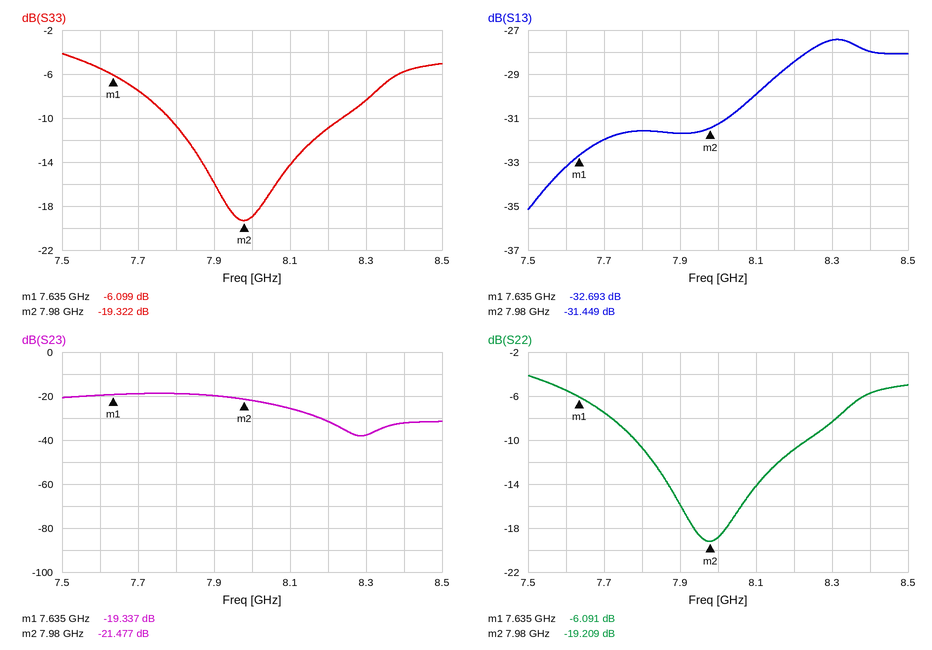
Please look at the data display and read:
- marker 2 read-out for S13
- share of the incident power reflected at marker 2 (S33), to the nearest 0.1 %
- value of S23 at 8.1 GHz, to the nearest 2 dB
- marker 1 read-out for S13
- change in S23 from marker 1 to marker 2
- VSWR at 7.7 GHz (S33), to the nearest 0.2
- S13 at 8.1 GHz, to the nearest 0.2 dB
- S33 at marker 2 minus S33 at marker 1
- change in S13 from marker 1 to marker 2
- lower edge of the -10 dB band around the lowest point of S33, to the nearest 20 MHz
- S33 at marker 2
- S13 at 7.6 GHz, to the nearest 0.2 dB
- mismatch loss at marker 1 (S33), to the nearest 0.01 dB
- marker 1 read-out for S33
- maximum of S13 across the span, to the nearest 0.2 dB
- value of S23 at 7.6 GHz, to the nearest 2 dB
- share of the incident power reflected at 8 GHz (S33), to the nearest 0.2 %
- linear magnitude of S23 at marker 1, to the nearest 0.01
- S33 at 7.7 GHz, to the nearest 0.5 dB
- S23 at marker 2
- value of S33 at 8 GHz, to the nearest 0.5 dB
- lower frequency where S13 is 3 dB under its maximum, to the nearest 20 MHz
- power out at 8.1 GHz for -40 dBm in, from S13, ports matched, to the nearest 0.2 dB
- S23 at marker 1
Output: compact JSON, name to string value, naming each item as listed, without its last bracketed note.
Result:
{"marker 2 read-out for S13": "-31.449 dB", "share of the incident power reflected at marker 2 (S33), to the nearest 0.1 %": "1.2 %", "value of S23 at 8.1 GHz, to the nearest 2 dB": "-26 dB", "marker 1 read-out for S13": "-32.693 dB", "change in S23 from marker 1 to marker 2": "-2.140 dB", "VSWR at 7.7 GHz (S33), to the nearest 0.2": "2.4", "S13 at 8.1 GHz, to the nearest 0.2 dB": "-30.0 dB", "S33 at marker 2 minus S33 at marker 1": "-13.223 dB", "change in S13 from marker 1 to marker 2": "1.244 dB", "lower edge of the -10 dB band around the lowest point of S33, to the nearest 20 MHz": "7.78 GHz", "S33 at marker 2": "-19.322 dB", "S13 at 7.6 GHz, to the nearest 0.2 dB": "-33.2 dB", "mismatch loss at marker 1 (S33), to the nearest 0.01 dB": "1.22 dB", "marker 1 read-out for S33": "-6.099 dB", "maximum of S13 across the span, to the nearest 0.2 dB": "-27.4 dB", "value of S23 at 7.6 GHz, to the nearest 2 dB": "-20 dB", "share of the incident power reflected at 8 GHz (S33), to the nearest 0.2 %": "1.2 %", "linear magnitude of S23 at marker 1, to the nearest 0.01": "0.11", "S33 at 7.7 GHz, to the nearest 0.5 dB": "-7.5 dB", "S23 at marker 2": "-21.477 dB", "value of S33 at 8 GHz, to the nearest 0.5 dB": "-19.0 dB", "lower frequency where S13 is 3 dB under its maximum, to the nearest 20 MHz": "8.06 GHz", "power out at 8.1 GHz for -40 dBm in, from S13, ports matched, to the nearest 0.2 dB": "-70.0 dBm", "S23 at marker 1": "-19.337 dB"}
